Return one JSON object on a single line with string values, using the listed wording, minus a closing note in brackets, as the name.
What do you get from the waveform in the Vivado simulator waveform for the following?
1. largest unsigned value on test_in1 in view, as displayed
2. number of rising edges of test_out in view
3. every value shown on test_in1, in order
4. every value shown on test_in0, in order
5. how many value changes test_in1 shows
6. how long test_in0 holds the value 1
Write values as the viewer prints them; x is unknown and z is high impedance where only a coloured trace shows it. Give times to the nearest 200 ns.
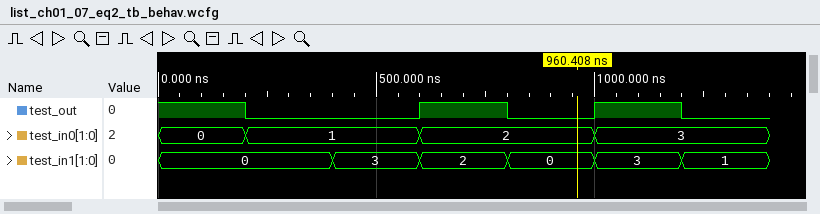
{"largest unsigned value on test_in1 in view, as displayed": "3", "number of rising edges of test_out in view": "2", "every value shown on test_in1, in order": "0, 3, 2, 0, 3, 1", "every value shown on test_in0, in order": "0, 1, 2, 3", "how many value changes test_in1 shows": "5", "how long test_in0 holds the value 1": "400 ns"}
